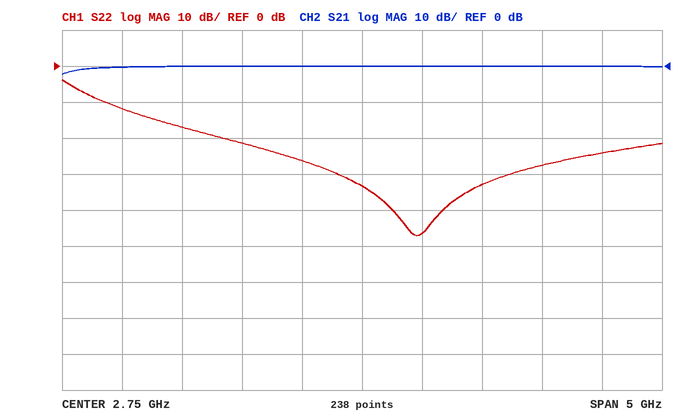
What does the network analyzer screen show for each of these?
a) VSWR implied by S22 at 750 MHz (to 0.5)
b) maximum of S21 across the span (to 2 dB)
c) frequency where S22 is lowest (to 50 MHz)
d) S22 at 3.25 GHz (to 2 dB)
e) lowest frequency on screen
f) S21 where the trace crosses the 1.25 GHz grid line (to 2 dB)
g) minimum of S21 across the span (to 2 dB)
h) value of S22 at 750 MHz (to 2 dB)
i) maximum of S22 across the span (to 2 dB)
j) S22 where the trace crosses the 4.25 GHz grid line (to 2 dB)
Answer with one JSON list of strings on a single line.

["1.5", "0 dB", "3.20 GHz", "-46 dB", "250 MHz", "0 dB", "-2 dB", "-12 dB", "-4 dB", "-28 dB"]
